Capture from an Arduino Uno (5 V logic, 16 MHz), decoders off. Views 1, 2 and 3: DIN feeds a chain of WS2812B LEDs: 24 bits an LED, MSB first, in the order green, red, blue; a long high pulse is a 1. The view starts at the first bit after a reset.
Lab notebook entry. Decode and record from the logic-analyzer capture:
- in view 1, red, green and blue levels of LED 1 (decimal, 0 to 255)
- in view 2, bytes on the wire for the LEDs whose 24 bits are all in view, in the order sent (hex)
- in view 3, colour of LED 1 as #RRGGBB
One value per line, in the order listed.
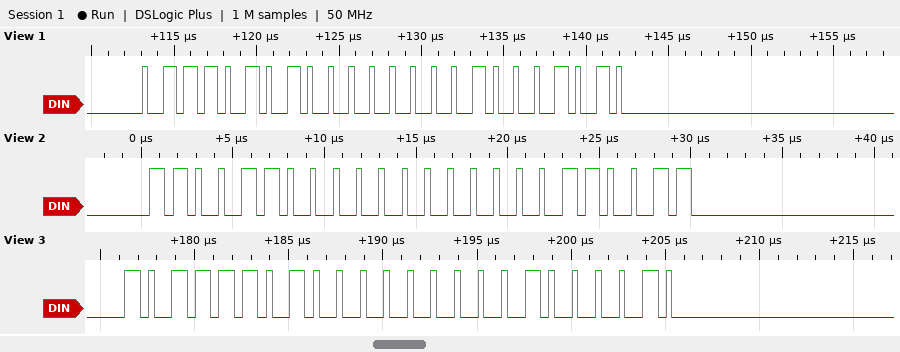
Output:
0, 117, 138
CC 00 33
#00BD42
